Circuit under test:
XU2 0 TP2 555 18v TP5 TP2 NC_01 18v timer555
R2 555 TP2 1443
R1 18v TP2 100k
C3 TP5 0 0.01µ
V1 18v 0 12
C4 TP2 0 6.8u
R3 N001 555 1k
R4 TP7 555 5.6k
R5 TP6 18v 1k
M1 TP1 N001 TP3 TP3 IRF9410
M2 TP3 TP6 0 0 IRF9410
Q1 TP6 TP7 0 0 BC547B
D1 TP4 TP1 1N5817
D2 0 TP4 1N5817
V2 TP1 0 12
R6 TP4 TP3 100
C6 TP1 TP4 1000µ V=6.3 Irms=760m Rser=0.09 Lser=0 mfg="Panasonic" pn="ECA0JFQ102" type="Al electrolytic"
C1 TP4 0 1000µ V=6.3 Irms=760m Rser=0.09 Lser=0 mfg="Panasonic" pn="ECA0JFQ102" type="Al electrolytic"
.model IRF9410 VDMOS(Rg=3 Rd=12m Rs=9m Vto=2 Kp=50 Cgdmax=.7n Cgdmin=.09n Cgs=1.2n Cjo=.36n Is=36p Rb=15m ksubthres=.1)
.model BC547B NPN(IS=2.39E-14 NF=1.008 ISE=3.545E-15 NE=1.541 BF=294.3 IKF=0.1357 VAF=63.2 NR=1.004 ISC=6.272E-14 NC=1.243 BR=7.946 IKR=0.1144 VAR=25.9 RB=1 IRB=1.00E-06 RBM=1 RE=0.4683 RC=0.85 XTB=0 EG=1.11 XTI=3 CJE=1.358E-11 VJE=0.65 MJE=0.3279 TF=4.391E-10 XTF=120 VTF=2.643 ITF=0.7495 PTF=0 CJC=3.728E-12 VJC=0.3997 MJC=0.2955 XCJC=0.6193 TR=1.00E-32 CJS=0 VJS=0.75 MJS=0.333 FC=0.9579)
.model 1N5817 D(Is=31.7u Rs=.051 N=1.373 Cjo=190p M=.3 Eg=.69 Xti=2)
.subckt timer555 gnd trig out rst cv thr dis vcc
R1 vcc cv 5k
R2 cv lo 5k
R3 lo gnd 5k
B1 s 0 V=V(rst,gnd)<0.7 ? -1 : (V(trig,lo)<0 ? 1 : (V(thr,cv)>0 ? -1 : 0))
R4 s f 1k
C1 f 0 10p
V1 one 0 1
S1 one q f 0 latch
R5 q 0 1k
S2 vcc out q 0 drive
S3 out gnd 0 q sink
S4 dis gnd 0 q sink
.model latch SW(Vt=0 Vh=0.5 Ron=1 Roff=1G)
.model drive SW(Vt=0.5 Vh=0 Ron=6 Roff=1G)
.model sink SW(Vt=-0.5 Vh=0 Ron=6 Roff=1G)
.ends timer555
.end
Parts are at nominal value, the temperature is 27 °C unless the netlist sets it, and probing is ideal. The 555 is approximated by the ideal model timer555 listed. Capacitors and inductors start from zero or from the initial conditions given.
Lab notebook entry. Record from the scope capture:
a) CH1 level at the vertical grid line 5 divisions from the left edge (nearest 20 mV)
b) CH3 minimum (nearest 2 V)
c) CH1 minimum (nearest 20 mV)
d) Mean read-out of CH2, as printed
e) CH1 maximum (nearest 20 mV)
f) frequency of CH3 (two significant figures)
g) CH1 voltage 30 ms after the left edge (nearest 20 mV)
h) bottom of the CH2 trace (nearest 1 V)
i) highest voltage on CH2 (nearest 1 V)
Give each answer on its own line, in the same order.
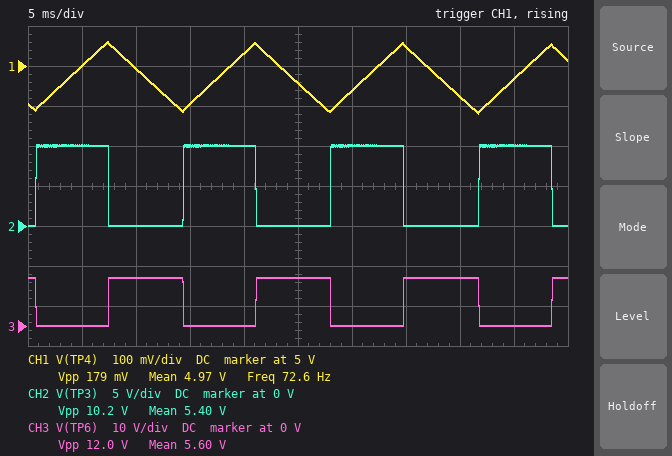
4.96 V
0 V
4.88 V
5.40 V
5.06 V
73 Hz
4.94 V
0 V
10 V
